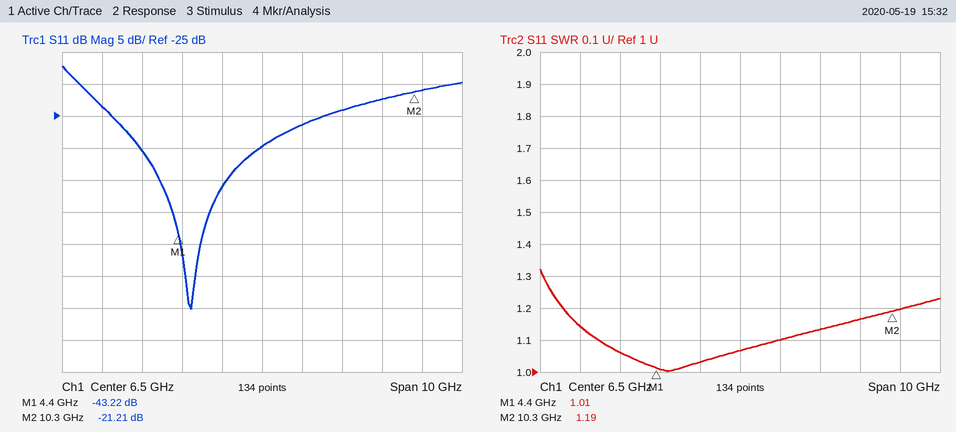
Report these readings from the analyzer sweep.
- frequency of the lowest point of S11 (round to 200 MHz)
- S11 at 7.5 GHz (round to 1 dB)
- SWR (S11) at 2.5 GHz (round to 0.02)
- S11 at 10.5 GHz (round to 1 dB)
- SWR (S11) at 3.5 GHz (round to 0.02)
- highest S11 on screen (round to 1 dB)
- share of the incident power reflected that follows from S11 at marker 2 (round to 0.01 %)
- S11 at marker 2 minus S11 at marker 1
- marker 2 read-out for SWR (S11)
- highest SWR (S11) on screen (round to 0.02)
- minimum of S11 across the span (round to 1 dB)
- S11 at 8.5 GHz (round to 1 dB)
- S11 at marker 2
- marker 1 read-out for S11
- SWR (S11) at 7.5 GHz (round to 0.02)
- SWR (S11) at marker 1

4.8 GHz
-26 dB
1.14
-21 dB
1.06
-17 dB
0.76 %
22.01 dB
1.19
1.32
-55 dB
-24 dB
-21.21 dB
-43.22 dB
1.10
1.01
